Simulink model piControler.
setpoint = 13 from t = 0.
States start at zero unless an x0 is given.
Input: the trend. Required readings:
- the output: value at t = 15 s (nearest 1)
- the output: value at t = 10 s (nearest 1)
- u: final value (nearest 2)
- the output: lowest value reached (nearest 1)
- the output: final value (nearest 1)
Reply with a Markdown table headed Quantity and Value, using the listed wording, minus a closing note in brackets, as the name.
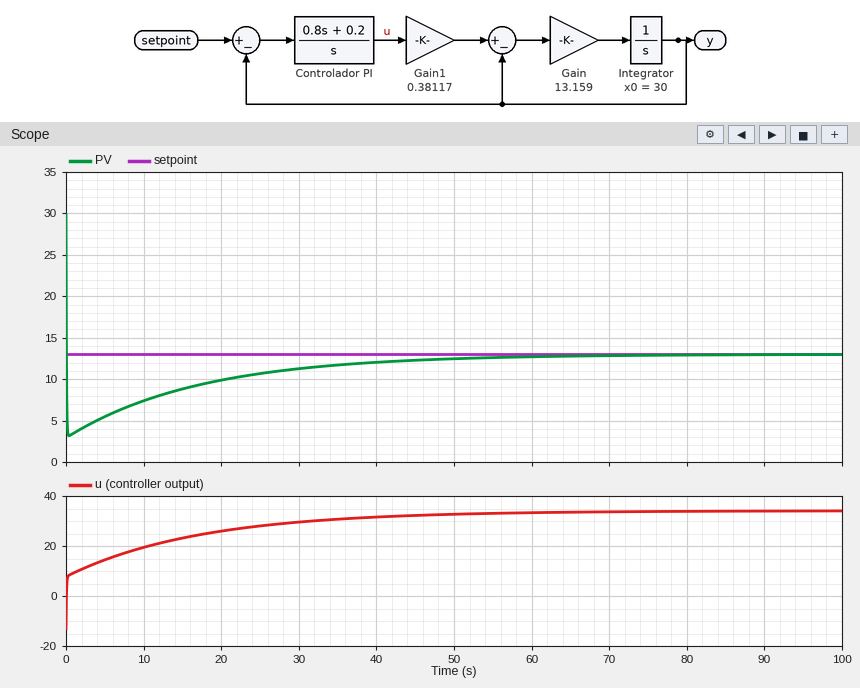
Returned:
| Quantity | Value |
|---|---|
| the output: value at t = 15 s | 9 |
| the output: value at t = 10 s | 7 |
| u: final value | 34 |
| the output: lowest value reached | 3 |
| the output: final value | 13 |
